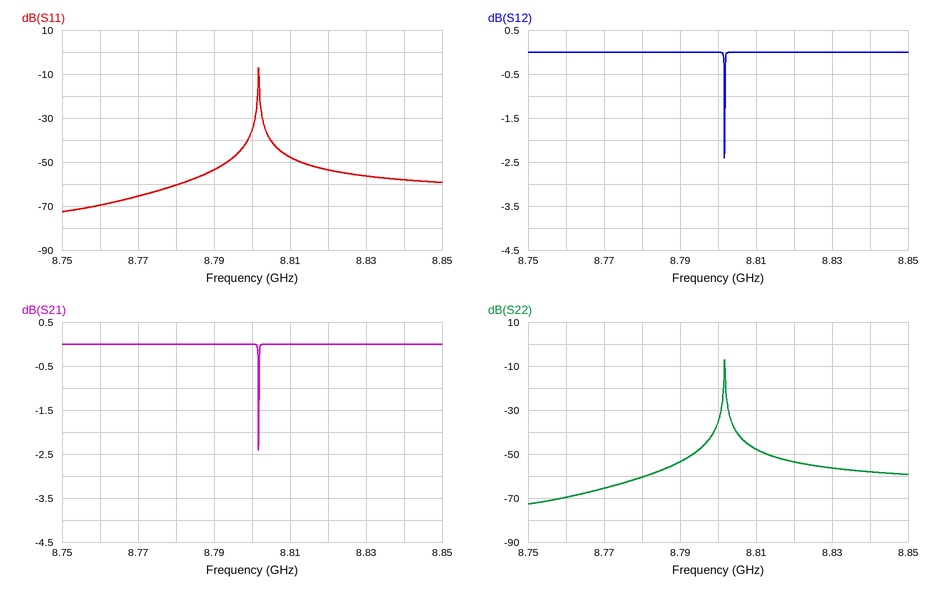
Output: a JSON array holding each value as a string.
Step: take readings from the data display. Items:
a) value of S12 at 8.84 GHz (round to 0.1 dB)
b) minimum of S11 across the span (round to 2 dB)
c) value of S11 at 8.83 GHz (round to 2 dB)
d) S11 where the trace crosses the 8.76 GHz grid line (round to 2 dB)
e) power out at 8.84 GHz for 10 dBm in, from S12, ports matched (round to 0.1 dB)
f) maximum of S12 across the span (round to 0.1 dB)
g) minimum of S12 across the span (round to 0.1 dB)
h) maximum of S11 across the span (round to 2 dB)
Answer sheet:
["0.0 dB", "-72 dB", "-56 dB", "-70 dB", "10.0 dBm", "0.0 dB", "-2.4 dB", "-8 dB"]
